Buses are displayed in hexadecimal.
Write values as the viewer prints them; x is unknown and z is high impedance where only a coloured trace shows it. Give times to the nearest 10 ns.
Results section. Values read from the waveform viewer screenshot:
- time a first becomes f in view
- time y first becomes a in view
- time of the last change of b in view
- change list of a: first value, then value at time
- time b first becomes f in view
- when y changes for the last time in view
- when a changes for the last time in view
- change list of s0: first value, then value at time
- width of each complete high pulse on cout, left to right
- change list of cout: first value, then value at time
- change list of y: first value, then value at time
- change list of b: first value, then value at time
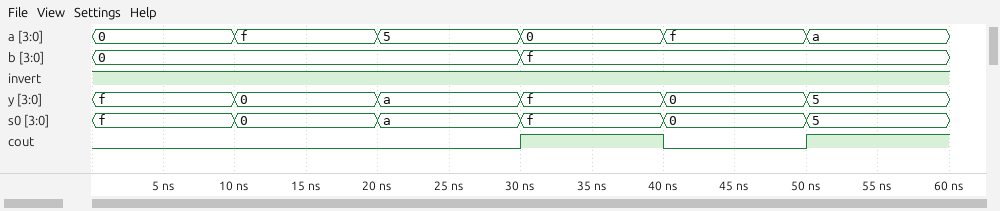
10 ns
20 ns
30 ns
0, f at 10 ns, 5 at 20 ns, 0 at 30 ns, f at 40 ns, a at 50 ns
30 ns
50 ns
50 ns
f, 0 at 10 ns, a at 20 ns, f at 30 ns, 0 at 40 ns, 5 at 50 ns
10 ns
0, 1 at 30 ns, 0 at 40 ns, 1 at 50 ns
f, 0 at 10 ns, a at 20 ns, f at 30 ns, 0 at 40 ns, 5 at 50 ns
0, f at 30 ns
